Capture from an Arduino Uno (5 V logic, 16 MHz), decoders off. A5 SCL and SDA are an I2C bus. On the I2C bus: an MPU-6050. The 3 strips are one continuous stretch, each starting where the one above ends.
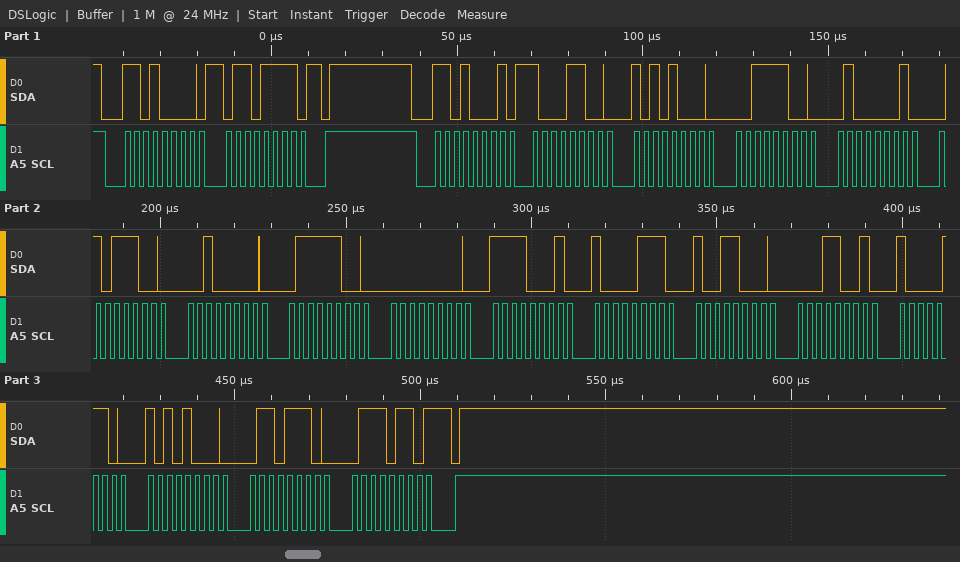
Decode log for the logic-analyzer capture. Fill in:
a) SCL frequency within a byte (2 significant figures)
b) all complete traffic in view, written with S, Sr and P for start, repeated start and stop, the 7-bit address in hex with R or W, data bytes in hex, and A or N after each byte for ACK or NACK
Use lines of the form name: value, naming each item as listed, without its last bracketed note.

SCL frequency within a byte: 400 kHz
all complete traffic in view, written with S, Sr and P for start, repeated start and stop, the 7-bit address in hex with R or W, data bytes in hex, and A or N after each byte for ACK or NACK: S 68W A 6F A P S 68R A 8C A A8 A 3C A 41 A 5C A 20 A 7C A 00 A F1 A 87 A 98 A 19 A 86 A A8 A 6E A 76 N P
